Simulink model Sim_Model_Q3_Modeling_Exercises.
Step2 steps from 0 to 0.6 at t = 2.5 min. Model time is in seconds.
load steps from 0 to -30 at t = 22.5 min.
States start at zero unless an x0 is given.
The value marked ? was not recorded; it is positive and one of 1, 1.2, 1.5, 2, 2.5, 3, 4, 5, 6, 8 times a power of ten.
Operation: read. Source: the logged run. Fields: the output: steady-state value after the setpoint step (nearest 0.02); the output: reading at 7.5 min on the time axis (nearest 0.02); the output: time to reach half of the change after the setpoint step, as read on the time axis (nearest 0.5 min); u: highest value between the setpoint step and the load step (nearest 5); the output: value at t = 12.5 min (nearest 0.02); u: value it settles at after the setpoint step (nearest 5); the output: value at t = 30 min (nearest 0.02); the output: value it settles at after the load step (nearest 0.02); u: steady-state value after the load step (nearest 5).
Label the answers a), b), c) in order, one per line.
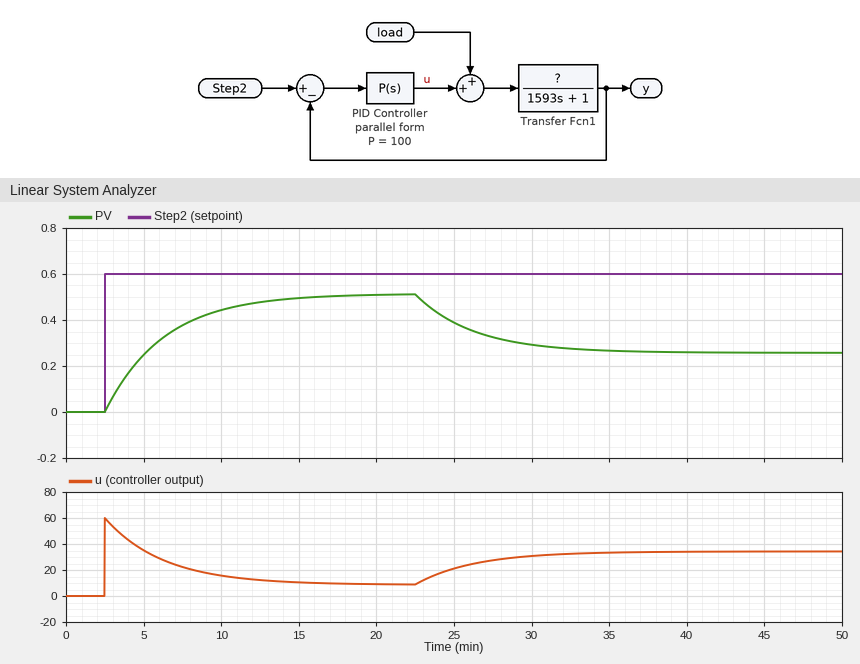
a) 0.52
b) 0.38
c) 5.0 min
d) 60
e) 0.48
f) 10
g) 0.30
h) 0.26
i) 35
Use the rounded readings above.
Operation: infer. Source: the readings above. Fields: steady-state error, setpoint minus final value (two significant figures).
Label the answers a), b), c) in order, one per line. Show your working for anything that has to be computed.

a) 0.6 - 0.52 = 0.080
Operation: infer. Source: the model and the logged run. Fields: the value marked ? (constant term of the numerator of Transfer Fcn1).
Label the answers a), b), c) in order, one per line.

a) 0.06
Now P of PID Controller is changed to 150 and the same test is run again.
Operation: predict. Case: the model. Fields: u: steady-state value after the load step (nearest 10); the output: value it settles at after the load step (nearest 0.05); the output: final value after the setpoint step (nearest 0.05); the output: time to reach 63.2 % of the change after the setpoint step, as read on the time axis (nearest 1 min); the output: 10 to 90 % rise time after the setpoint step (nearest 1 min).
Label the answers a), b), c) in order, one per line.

a) 40
b) 0.35
c) 0.55
d) 5 min
e) 6 min
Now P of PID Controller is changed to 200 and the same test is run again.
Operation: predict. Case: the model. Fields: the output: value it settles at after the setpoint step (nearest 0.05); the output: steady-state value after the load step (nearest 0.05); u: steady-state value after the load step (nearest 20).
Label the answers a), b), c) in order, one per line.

a) 0.55
b) 0.40
c) 40
